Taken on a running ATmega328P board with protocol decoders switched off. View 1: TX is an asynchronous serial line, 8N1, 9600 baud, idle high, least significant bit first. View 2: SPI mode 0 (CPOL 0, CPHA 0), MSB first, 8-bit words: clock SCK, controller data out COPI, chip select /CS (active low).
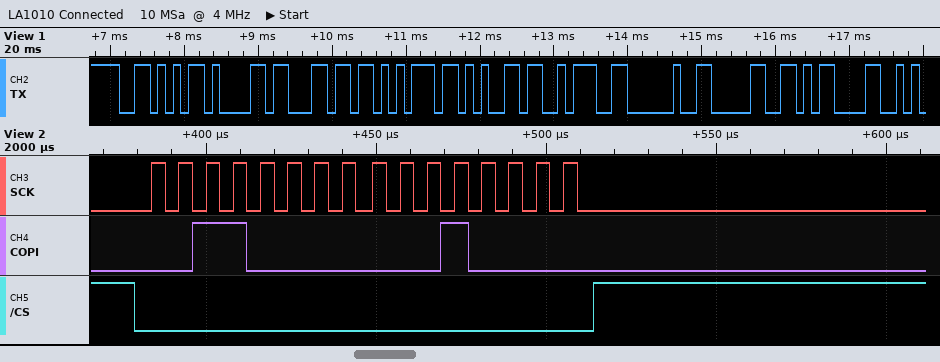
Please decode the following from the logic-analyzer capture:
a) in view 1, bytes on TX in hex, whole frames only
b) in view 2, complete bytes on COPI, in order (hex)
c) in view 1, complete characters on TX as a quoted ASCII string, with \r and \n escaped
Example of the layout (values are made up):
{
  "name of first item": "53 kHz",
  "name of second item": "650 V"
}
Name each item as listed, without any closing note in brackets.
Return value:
{
  "in view 1, bytes on TX in hex, whole frames only": "56 61 6C 75 65 3A 20 30 0D",
  "in view 2, complete bytes on COPI, in order": "30 10",
  "in view 1, complete characters on TX as a quoted ASCII string, with \\r and \\n escaped": "\"Value: 0\\r\""
}
